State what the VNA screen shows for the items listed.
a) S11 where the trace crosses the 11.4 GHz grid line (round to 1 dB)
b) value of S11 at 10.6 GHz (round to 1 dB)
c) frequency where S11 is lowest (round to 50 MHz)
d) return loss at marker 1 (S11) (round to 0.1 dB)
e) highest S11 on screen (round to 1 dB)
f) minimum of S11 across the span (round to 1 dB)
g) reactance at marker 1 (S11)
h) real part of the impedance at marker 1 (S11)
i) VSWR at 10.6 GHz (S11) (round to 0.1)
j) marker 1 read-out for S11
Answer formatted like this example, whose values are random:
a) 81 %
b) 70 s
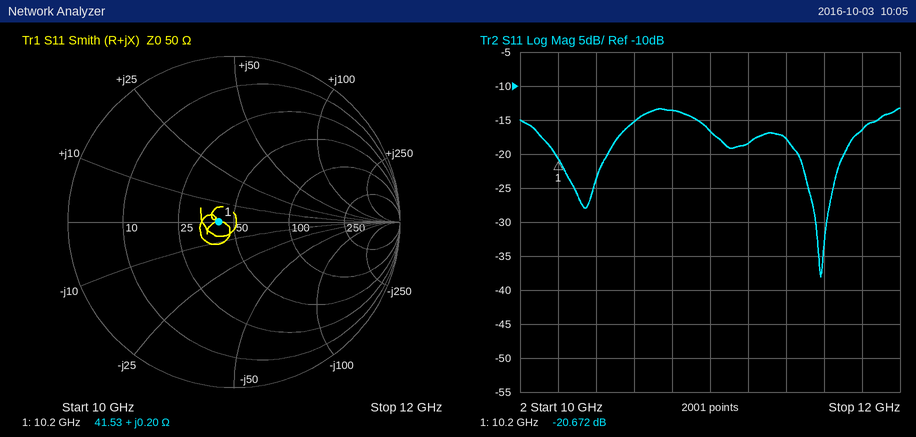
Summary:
a) -18 dB
b) -15 dB
c) 11.60 GHz
d) 20.7 dB
e) -13 dB
f) -38 dB
g) +0.20 Ω
h) 41.53 Ω
i) 1.4
j) -20.672 dB
